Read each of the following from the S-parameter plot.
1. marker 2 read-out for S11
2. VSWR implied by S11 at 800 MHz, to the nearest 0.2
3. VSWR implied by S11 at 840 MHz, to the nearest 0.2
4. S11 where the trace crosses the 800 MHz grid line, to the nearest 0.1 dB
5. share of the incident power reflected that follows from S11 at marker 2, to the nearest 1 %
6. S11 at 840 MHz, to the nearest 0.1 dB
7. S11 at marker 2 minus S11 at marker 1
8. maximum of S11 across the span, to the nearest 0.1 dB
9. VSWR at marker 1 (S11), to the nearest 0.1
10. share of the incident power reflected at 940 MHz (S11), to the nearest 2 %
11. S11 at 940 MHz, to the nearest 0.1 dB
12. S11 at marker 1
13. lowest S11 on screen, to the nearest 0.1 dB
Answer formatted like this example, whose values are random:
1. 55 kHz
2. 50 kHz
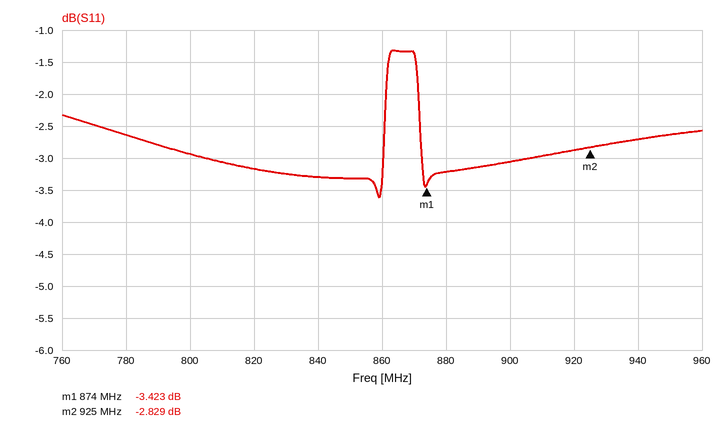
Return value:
1. -2.829 dB
2. 6.0
3. 5.4
4. -2.9 dB
5. 52 %
6. -3.3 dB
7. 0.594 dB
8. -1.3 dB
9. 5.1
10. 54 %
11. -2.7 dB
12. -3.423 dB
13. -3.6 dB
